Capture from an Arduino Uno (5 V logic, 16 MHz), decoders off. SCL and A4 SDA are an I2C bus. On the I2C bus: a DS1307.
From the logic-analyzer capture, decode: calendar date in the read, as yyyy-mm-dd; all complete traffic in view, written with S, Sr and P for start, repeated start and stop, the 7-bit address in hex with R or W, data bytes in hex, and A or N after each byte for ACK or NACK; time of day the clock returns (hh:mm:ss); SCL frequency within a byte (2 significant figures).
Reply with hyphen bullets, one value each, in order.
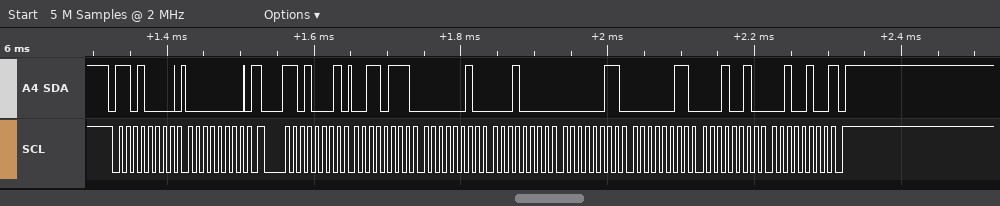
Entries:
- 2024-12-03
- S 68W A 00 A Sr 68R A 37 A 02 A 10 A 03 A 03 A 12 A 24 N P
- 10:02:37
- 100 kHz
